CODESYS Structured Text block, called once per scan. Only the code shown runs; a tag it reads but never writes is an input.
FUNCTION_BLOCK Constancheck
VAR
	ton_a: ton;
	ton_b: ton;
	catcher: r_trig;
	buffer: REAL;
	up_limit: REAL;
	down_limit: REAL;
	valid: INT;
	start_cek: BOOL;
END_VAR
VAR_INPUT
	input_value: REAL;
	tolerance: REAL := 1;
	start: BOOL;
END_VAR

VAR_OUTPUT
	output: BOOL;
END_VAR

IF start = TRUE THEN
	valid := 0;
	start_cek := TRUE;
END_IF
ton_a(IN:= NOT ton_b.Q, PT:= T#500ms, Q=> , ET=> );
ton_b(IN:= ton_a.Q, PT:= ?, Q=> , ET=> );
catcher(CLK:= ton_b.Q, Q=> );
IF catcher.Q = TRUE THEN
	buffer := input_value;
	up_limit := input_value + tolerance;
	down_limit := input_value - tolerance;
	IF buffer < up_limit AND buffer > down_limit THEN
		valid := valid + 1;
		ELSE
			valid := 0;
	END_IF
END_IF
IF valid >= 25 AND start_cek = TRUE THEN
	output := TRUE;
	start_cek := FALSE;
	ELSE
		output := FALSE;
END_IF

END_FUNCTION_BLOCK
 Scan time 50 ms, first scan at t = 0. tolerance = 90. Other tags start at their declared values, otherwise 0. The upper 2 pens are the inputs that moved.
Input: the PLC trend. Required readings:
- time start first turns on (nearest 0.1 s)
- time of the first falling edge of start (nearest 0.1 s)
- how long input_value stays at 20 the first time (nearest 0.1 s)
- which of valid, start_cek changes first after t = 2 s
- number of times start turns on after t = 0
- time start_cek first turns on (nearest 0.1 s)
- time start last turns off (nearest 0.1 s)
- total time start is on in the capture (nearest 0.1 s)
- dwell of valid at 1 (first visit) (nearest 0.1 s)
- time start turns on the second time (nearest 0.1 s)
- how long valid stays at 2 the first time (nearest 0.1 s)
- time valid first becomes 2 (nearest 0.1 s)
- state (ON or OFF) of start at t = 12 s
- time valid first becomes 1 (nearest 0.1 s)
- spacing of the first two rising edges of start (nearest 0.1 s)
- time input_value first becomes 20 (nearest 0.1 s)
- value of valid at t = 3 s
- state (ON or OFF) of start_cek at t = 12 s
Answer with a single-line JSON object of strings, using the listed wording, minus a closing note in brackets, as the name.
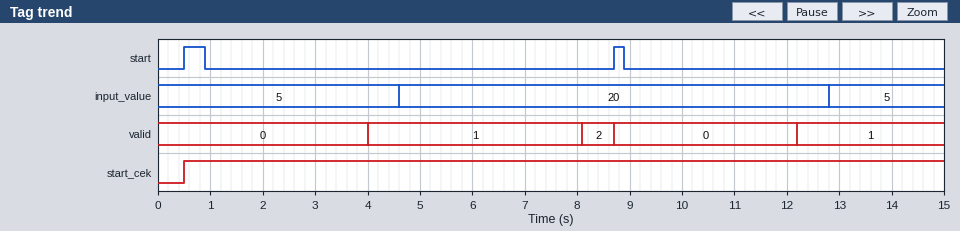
{"time start first turns on": "0.5 s", "time of the first falling edge of start": "0.9 s", "how long input_value stays at 20 the first time": "8.2 s", "which of valid, start_cek changes first after t = 2 s": "valid", "number of times start turns on after t = 0": "2", "time start_cek first turns on": "0.5 s", "time start last turns off": "8.9 s", "total time start is on in the capture": "0.6 s", "dwell of valid at 1 (first visit)": "4.1 s", "time start turns on the second time": "8.7 s", "how long valid stays at 2 the first time": "0.6 s", "time valid first becomes 2": "8.1 s", "state (ON or OFF) of start at t = 12 s": "OFF", "time valid first becomes 1": "4.0 s", "spacing of the first two rising edges of start": "8.2 s", "time input_value first becomes 20": "4.6 s", "value of valid at t = 3 s": "0", "state (ON or OFF) of start_cek at t = 12 s": "ON"}
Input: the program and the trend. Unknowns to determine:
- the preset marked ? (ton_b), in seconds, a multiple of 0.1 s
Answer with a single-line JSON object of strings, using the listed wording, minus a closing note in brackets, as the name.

{"the preset marked ? (ton_b), in seconds, a multiple of 0.1 s": "3.5 s"}
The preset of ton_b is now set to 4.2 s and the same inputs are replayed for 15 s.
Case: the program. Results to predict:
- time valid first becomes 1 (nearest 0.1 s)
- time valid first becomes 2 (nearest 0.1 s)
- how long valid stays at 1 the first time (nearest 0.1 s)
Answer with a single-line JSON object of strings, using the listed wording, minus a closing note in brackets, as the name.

{"time valid first becomes 1": "4.7 s", "time valid first becomes 2": "14.3 s", "how long valid stays at 1 the first time": "4.0 s"}
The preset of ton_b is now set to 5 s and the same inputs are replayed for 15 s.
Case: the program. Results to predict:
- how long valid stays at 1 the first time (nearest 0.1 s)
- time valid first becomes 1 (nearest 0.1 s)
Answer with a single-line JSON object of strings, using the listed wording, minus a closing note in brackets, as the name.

{"how long valid stays at 1 the first time": "3.2 s", "time valid first becomes 1": "5.5 s"}
